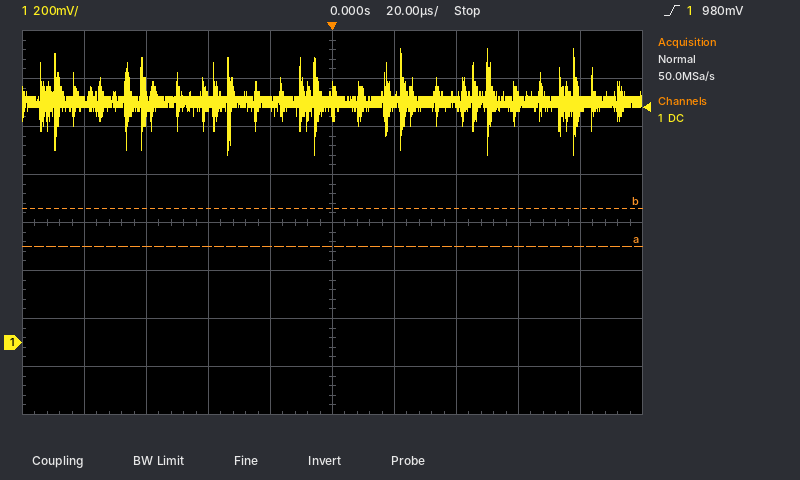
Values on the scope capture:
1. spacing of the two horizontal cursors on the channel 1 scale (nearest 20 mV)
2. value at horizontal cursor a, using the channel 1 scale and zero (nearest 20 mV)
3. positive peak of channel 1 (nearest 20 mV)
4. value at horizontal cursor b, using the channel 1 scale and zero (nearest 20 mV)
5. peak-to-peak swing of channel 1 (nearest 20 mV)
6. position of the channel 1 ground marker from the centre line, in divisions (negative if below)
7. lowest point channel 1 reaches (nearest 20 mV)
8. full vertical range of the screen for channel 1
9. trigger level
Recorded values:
160 mV
400 mV
1.22 V
560 mV
440 mV
-2.5 div
780 mV
1.6 V
980 mV
